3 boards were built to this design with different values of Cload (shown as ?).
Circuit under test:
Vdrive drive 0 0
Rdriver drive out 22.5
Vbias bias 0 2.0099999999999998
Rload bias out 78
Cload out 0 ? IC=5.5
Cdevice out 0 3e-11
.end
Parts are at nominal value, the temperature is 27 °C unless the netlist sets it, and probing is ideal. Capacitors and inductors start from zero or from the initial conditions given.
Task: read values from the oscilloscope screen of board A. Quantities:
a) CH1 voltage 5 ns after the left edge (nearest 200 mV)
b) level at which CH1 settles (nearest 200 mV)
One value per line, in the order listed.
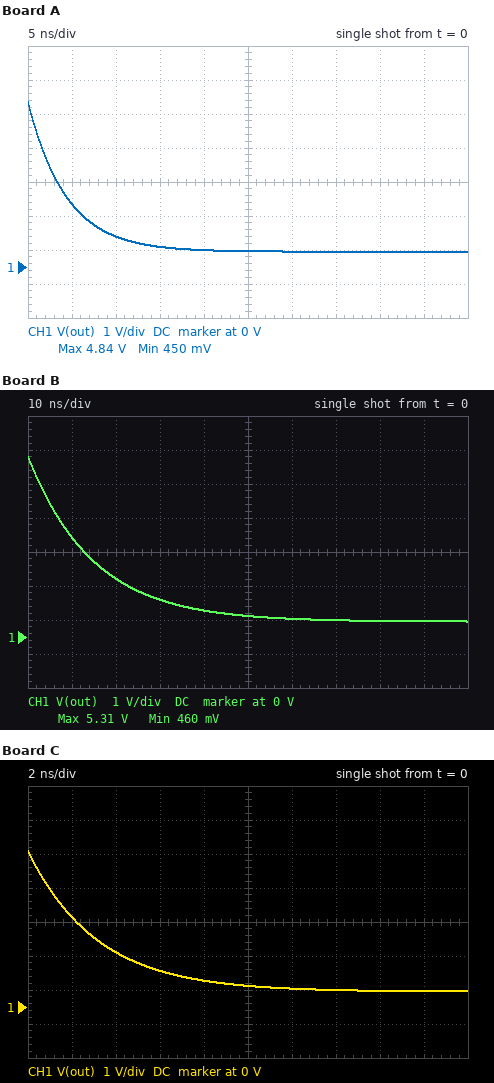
1.8 V
400 mV
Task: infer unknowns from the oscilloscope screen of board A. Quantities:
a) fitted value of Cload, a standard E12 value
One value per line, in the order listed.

220 pF
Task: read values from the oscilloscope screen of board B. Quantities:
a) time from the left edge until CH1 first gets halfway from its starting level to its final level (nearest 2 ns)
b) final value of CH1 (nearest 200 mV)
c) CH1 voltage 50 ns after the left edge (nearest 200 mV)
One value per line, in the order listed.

10 ns
400 mV
600 mV
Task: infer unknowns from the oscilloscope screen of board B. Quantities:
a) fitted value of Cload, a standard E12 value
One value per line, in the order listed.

820 pF
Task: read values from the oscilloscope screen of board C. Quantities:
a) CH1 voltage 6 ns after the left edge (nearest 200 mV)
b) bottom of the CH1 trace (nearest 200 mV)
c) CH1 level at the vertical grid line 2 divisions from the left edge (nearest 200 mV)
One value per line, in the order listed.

1.0 V
400 mV
1.6 V
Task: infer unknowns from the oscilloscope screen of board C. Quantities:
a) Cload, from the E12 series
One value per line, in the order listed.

150 pF
